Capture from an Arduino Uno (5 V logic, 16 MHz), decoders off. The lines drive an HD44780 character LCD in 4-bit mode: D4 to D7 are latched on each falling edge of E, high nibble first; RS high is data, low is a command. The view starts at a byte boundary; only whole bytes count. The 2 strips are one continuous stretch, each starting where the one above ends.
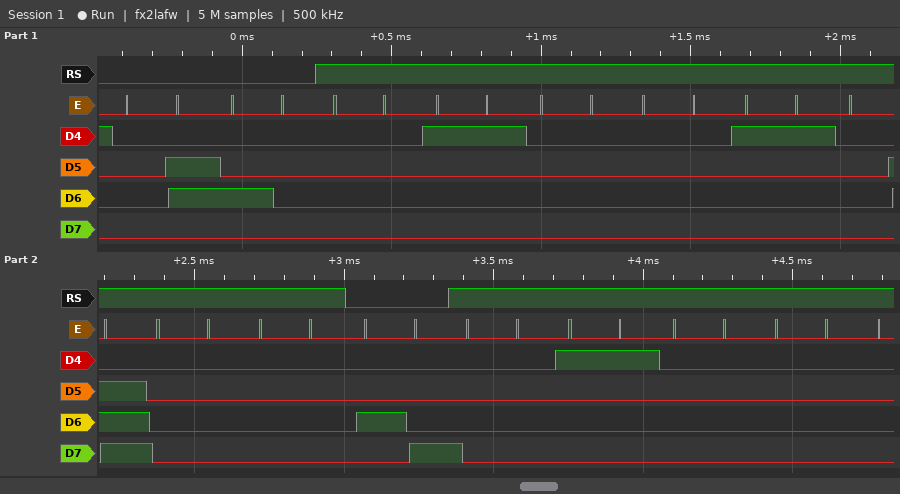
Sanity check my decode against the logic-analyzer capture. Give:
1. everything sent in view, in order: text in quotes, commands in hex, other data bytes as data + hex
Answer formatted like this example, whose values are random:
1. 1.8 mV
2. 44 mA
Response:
1. 0x06 0x40 data 00 11 00 00 11 0E 00 00 0x48 data 00 11 00 00
